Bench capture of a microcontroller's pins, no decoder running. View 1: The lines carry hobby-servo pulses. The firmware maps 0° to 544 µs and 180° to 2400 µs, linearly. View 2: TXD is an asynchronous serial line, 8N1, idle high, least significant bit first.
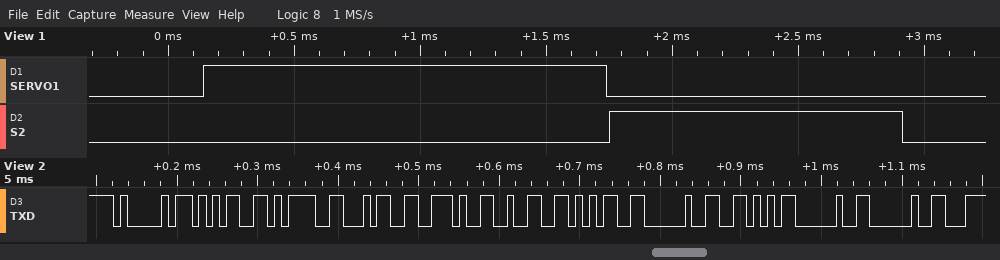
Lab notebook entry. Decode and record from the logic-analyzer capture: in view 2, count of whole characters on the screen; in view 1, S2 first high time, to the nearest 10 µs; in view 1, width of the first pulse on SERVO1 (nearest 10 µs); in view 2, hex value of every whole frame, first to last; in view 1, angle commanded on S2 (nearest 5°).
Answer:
11
1160 µs
1600 µs
41 35 3D 34 2E 32 35 20 56 20 20
60°
